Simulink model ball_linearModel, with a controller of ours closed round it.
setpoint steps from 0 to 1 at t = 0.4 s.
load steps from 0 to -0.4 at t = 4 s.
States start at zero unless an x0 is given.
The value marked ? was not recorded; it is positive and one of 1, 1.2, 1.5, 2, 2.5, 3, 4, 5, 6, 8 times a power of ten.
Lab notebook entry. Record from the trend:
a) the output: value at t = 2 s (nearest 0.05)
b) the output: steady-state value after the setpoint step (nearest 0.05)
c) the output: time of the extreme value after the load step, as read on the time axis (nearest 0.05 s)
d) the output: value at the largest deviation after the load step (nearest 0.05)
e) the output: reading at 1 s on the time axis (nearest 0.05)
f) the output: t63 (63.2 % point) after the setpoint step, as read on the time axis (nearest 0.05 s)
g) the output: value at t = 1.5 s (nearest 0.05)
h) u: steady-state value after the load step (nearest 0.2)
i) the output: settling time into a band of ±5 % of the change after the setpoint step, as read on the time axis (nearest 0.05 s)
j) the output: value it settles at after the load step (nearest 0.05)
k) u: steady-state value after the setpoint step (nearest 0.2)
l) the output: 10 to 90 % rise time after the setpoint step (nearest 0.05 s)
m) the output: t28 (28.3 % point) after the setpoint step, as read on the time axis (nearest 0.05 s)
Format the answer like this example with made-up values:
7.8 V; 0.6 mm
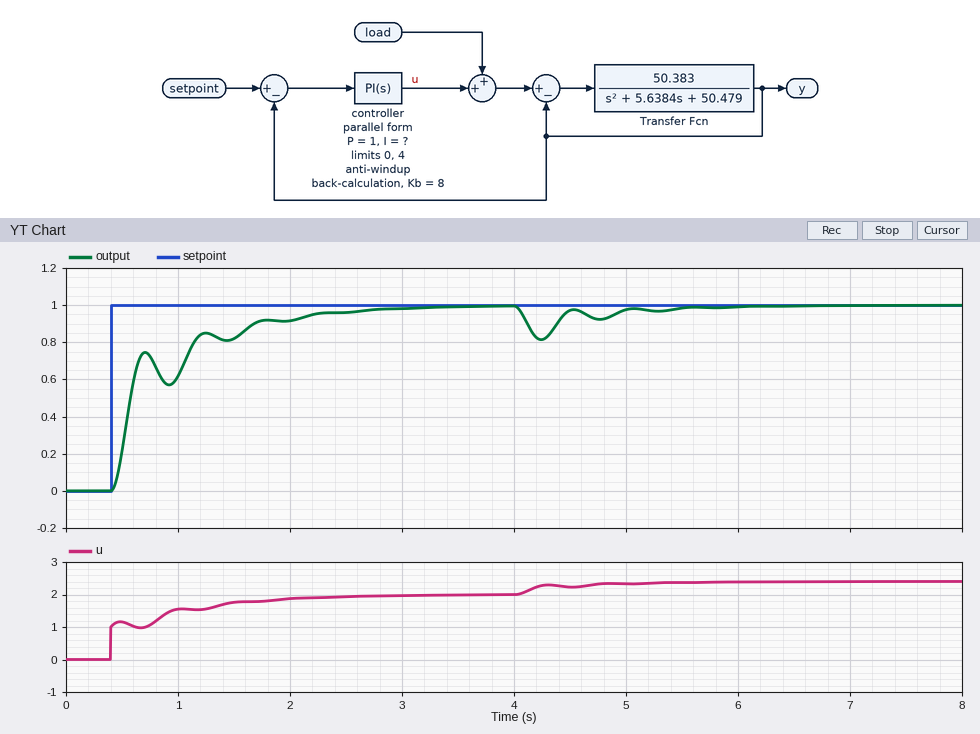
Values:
0.90; 1.00; 4.25 s; 0.80; 0.60; 0.60 s; 0.80; 2.4; 2.20 s; 1.00; 2.0; 1.20 s; 0.50 s
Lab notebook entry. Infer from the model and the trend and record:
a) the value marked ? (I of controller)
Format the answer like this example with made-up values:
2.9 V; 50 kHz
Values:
4
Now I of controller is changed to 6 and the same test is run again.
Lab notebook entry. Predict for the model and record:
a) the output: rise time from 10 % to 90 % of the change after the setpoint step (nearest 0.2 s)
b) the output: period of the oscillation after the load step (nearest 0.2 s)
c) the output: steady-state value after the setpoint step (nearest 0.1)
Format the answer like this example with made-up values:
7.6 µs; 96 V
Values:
0.6 s; 0.6 s; 1.0
